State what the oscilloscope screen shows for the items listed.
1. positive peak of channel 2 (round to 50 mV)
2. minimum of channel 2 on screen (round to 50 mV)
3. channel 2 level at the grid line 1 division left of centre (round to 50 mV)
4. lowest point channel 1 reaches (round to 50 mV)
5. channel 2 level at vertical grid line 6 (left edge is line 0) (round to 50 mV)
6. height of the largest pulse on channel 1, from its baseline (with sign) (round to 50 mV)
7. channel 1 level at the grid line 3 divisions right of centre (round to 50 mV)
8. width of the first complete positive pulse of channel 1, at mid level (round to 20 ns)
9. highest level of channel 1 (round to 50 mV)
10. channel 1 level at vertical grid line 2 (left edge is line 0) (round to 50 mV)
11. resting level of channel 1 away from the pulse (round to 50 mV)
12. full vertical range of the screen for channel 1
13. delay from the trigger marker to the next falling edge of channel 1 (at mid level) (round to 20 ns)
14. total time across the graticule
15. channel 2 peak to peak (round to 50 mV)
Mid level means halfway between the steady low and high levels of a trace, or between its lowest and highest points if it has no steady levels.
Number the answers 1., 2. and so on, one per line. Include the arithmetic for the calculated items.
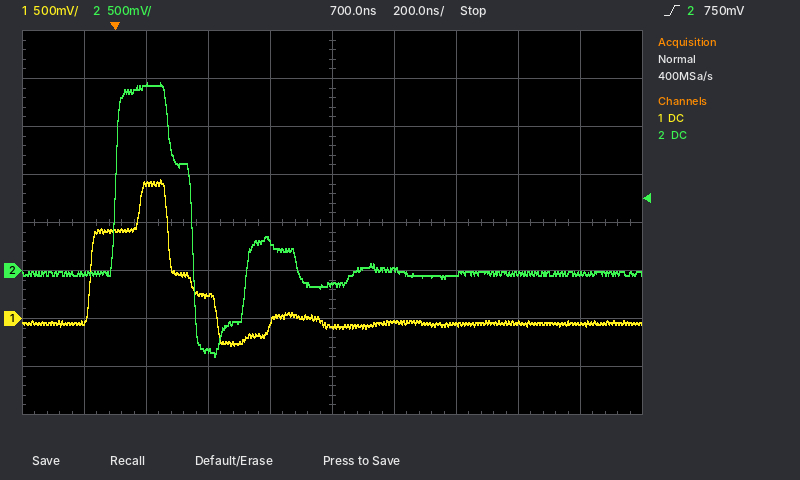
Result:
1. 1.95 V
2. -900 mV
3. 300 mV
4. -300 mV
5. 0 mV
6. 1.45 V − (-50 mV) = +1.50 V
7. -50 mV
8. 260 ns
9. 1.45 V
10. 1.40 V
11. -50 mV
12. 4 V
13. 180 ns
14. 2 µs
15. 1.95 V − (-900 mV) = 2.85 V
